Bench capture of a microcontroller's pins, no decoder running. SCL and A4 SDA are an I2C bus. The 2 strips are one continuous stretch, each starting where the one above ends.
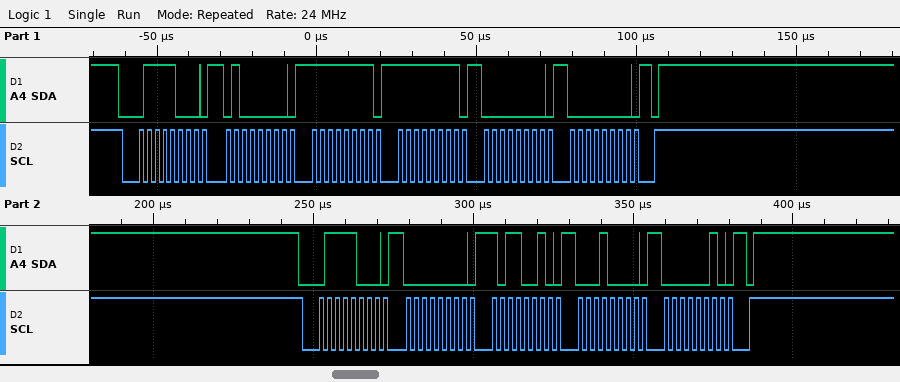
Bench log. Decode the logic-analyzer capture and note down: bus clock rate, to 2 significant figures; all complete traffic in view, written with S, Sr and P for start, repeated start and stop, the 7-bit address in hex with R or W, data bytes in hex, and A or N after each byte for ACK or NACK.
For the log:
400 kHz
S 3CW A 40 A FF A FF A 00 A 00 A P S 3CW A 00 A B2 A 10 A 02 A P
